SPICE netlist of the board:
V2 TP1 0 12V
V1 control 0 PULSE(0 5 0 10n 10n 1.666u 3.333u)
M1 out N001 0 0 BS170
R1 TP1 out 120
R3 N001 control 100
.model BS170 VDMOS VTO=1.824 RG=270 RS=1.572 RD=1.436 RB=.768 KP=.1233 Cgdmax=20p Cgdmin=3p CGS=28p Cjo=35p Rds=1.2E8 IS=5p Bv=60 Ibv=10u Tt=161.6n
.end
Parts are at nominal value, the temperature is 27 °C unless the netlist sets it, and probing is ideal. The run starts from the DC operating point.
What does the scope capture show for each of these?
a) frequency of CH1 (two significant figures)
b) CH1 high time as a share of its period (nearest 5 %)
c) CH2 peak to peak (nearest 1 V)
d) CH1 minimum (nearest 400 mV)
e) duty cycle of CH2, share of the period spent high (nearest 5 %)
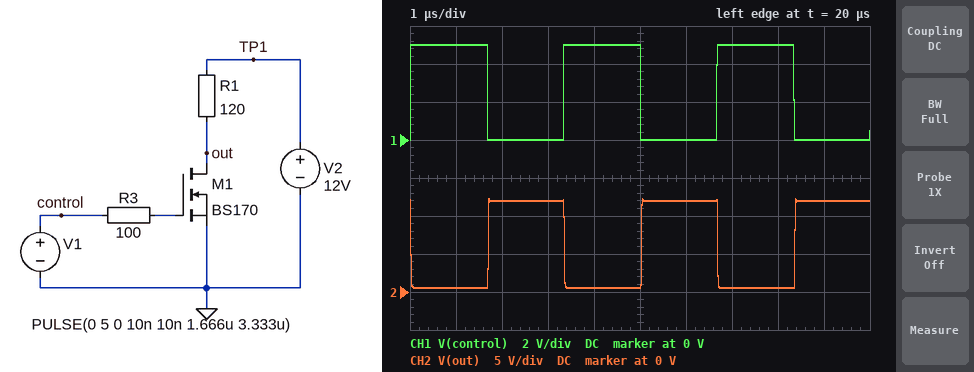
300 kHz
50 %
12 V
0 V
50 %
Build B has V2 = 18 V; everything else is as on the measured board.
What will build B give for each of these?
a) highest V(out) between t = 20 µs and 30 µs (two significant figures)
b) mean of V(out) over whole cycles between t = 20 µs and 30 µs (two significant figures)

18 V
9.4 V
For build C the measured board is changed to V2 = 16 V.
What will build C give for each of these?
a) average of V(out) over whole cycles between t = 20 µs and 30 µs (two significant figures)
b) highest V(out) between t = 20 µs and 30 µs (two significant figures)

8.3 V
16 V
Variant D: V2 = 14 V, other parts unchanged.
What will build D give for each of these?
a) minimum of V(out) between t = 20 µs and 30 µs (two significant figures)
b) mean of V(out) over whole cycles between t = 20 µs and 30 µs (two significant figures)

650 mV
7.3 V
